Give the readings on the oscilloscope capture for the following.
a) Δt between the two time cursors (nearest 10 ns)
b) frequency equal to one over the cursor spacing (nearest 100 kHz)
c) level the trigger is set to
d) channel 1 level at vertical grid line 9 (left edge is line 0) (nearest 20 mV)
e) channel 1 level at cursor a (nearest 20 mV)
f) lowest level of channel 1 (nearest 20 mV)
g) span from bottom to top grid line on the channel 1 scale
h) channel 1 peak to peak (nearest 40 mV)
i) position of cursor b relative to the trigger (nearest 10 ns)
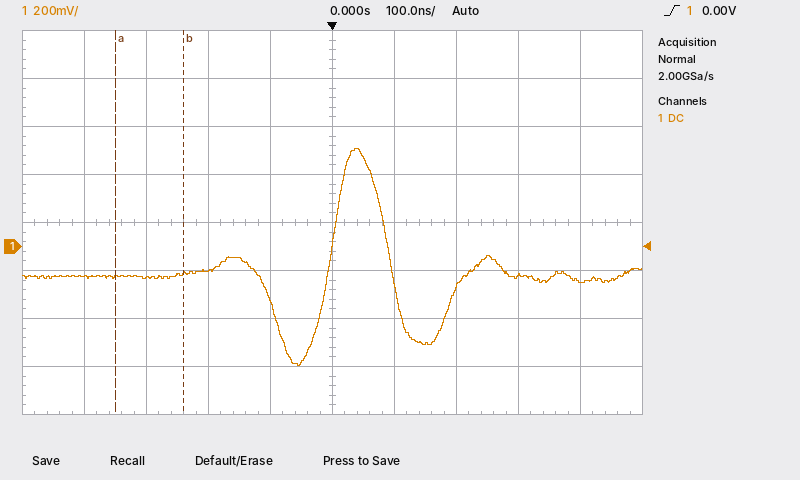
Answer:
110 ns
9.1 MHz
0.00 V
-140 mV
-120 mV
-500 mV
1.6 V
920 mV
-240 ns
